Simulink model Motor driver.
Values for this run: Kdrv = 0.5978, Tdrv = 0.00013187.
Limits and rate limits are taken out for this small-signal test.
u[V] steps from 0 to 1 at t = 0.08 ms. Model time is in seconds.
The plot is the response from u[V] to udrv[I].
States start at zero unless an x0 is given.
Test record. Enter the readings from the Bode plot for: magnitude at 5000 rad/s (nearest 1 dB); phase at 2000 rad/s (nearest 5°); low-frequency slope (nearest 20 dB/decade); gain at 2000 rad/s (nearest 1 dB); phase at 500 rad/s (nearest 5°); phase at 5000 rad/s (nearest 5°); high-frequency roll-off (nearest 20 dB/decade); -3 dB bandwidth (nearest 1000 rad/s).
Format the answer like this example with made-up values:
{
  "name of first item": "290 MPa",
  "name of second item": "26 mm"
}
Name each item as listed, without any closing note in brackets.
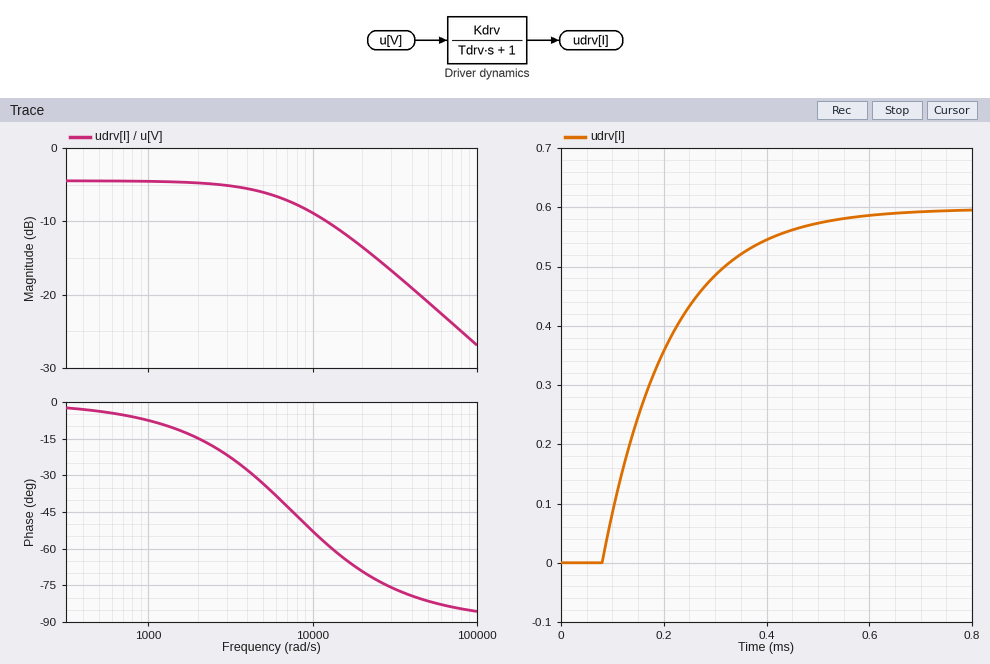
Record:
{
  "magnitude at 5000 rad/s": "-6 dB",
  "phase at 2000 rad/s": "-15°",
  "low-frequency slope": "0 dB/decade",
  "gain at 2000 rad/s": "-5 dB",
  "phase at 500 rad/s": "-5°",
  "phase at 5000 rad/s": "-35°",
  "high-frequency roll-off": "-20 dB/decade",
  "-3 dB bandwidth": "8000 rad/s"
}
